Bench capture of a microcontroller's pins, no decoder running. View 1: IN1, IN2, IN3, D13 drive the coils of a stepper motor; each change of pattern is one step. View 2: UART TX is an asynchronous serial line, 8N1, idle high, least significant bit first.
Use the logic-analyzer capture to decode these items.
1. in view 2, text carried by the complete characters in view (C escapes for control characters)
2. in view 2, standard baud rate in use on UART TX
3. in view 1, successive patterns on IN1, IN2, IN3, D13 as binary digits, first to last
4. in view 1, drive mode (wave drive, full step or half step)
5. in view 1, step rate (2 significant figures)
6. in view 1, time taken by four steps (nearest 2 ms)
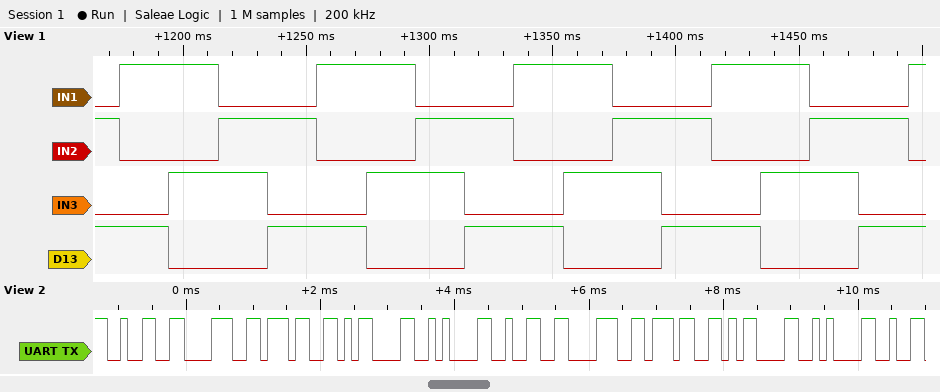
"287\r\n287\r\n"
9600 baud
0101 1001 1010 0110 0101 1001 1010 0110 0101 1001 1010 0110 0101 1001 1010 0110 0101 1001
full step
50 steps/s
80 ms
